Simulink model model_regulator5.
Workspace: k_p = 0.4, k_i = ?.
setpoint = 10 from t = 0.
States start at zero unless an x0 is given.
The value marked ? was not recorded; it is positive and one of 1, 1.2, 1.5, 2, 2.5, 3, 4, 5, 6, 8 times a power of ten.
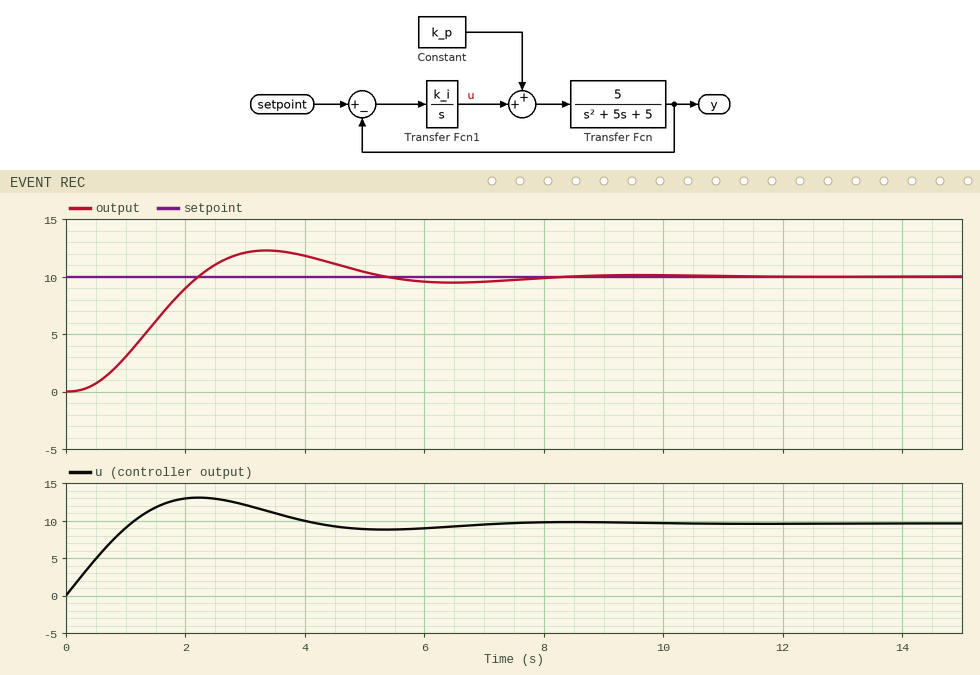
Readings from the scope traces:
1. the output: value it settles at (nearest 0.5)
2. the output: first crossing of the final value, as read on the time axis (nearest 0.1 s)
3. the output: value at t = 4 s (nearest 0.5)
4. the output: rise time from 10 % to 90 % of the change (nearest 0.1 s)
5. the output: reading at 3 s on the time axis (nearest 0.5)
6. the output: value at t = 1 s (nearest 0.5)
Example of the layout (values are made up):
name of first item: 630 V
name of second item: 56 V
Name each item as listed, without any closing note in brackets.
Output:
the output: value it settles at: 10.0
the output: first crossing of the final value, as read on the time axis: 2.2 s
the output: value at t = 4 s: 12.0
the output: rise time from 10 % to 90 % of the change: 1.4 s
the output: reading at 3 s on the time axis: 12.0
the output: value at t = 1 s: 3.0
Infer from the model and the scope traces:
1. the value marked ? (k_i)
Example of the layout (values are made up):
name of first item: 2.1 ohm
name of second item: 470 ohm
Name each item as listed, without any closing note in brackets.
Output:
the value marked ?: 1
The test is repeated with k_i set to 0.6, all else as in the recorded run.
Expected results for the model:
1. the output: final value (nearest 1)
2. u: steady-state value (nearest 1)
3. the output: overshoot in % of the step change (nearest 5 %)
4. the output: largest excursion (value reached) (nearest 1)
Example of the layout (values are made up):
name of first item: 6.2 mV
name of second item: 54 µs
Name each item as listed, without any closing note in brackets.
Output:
the output: final value: 10
u: steady-state value: 10
the output: overshoot in % of the step change: 10 %
the output: largest excursion (value reached): 11
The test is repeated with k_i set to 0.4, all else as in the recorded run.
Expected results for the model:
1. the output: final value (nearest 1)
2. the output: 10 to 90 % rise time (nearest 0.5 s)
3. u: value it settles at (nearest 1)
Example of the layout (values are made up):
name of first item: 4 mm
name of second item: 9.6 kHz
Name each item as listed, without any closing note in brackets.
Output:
the output: final value: 10
the output: 10 to 90 % rise time: 3.5 s
u: value it settles at: 10
